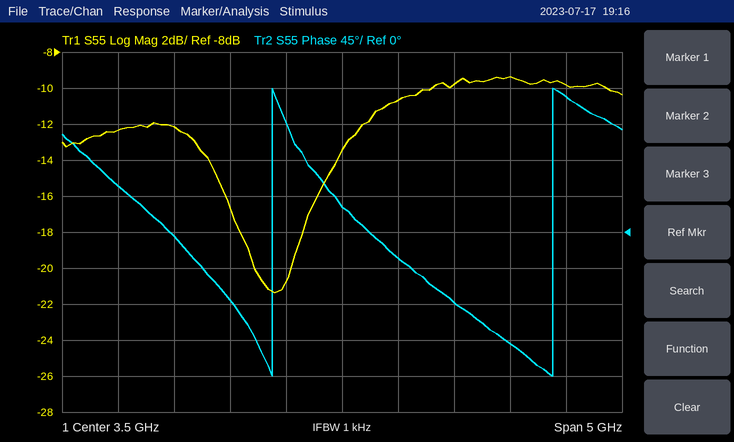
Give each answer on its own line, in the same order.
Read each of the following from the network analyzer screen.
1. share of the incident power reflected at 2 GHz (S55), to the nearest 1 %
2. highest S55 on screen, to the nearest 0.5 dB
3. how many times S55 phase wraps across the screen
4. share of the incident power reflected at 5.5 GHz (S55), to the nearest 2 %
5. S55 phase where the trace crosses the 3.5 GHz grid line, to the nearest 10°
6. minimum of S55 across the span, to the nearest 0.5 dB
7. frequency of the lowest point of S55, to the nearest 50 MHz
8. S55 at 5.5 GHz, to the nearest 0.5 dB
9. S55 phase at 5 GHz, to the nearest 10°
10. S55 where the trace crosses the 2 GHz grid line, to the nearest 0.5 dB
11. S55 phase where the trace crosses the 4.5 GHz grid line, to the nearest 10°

6 %
-9.5 dB
2
10 %
30°
-21.5 dB
2.90 GHz
-10.0 dB
-140°
-12.0 dB
-90°
